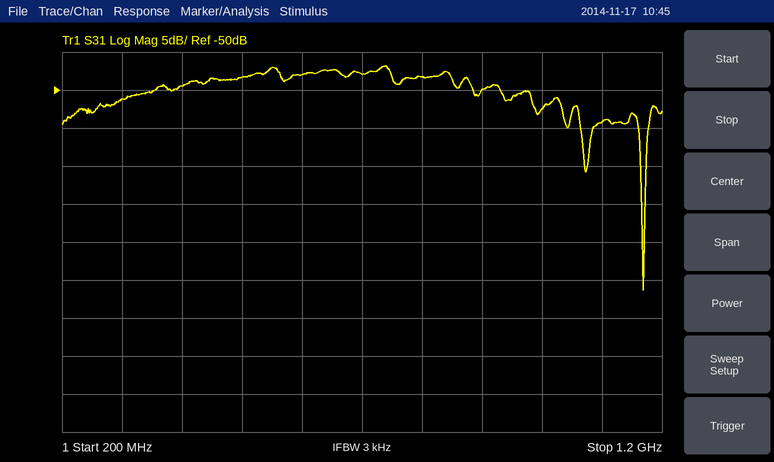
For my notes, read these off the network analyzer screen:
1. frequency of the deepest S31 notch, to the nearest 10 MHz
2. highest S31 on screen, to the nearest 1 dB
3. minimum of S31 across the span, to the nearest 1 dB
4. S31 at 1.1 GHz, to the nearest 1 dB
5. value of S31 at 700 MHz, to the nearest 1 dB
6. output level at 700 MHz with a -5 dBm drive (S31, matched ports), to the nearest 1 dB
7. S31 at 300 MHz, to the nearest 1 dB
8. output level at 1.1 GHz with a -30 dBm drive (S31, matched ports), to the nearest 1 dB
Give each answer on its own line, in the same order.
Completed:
1.17 GHz
-47 dB
-76 dB
-54 dB
-48 dB
-53 dBm
-51 dB
-84 dBm
